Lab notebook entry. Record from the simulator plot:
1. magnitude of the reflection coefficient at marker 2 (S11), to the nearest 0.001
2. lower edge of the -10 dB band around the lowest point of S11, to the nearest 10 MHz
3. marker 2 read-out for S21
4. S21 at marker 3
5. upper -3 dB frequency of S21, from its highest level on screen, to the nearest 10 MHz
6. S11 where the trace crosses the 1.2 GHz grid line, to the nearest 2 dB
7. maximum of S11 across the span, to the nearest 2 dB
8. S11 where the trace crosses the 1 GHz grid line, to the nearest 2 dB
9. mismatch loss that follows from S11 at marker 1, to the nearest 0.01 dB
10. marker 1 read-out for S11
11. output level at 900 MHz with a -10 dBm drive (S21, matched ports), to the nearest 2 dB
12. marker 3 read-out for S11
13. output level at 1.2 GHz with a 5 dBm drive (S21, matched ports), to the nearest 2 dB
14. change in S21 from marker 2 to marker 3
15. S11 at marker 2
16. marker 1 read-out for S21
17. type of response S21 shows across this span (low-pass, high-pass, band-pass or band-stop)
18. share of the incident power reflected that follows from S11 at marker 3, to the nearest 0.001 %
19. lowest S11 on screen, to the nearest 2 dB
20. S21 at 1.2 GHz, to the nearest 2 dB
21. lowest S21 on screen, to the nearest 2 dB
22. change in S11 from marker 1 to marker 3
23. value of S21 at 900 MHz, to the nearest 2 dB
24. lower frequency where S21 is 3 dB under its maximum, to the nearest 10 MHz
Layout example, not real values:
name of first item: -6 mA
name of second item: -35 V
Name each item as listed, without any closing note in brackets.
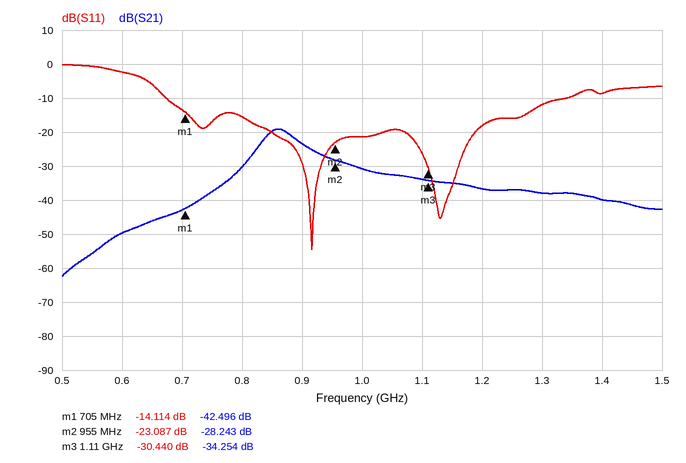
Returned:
magnitude of the reflection coefficient at marker 2 (S11), to the nearest 0.001: 0.070
lower edge of the -10 dB band around the lowest point of S11, to the nearest 10 MHz: 670 MHz
marker 2 read-out for S21: -28.243 dB
S21 at marker 3: -34.254 dB
upper -3 dB frequency of S21, from its highest level on screen, to the nearest 10 MHz: 890 MHz
S11 where the trace crosses the 1.2 GHz grid line, to the nearest 2 dB: -18 dB
maximum of S11 across the span, to the nearest 2 dB: 0 dB
S11 where the trace crosses the 1 GHz grid line, to the nearest 2 dB: -22 dB
mismatch loss that follows from S11 at marker 1, to the nearest 0.01 dB: 0.17 dB
marker 1 read-out for S11: -14.114 dB
output level at 900 MHz with a -10 dBm drive (S21, matched ports), to the nearest 2 dB: -34 dBm
marker 3 read-out for S11: -30.440 dB
output level at 1.2 GHz with a 5 dBm drive (S21, matched ports), to the nearest 2 dB: -32 dBm
change in S21 from marker 2 to marker 3: -6.011 dB
S11 at marker 2: -23.087 dB
marker 1 read-out for S21: -42.496 dB
type of response S21 shows across this span: band-pass
share of the incident power reflected that follows from S11 at marker 3, to the nearest 0.001 %: 0.090 %
lowest S11 on screen, to the nearest 2 dB: -54 dB
S21 at 1.2 GHz, to the nearest 2 dB: -36 dB
lowest S21 on screen, to the nearest 2 dB: -62 dB
change in S11 from marker 1 to marker 3: -16.326 dB
value of S21 at 900 MHz, to the nearest 2 dB: -24 dB
lower frequency where S21 is 3 dB under its maximum, to the nearest 10 MHz: 840 MHz
